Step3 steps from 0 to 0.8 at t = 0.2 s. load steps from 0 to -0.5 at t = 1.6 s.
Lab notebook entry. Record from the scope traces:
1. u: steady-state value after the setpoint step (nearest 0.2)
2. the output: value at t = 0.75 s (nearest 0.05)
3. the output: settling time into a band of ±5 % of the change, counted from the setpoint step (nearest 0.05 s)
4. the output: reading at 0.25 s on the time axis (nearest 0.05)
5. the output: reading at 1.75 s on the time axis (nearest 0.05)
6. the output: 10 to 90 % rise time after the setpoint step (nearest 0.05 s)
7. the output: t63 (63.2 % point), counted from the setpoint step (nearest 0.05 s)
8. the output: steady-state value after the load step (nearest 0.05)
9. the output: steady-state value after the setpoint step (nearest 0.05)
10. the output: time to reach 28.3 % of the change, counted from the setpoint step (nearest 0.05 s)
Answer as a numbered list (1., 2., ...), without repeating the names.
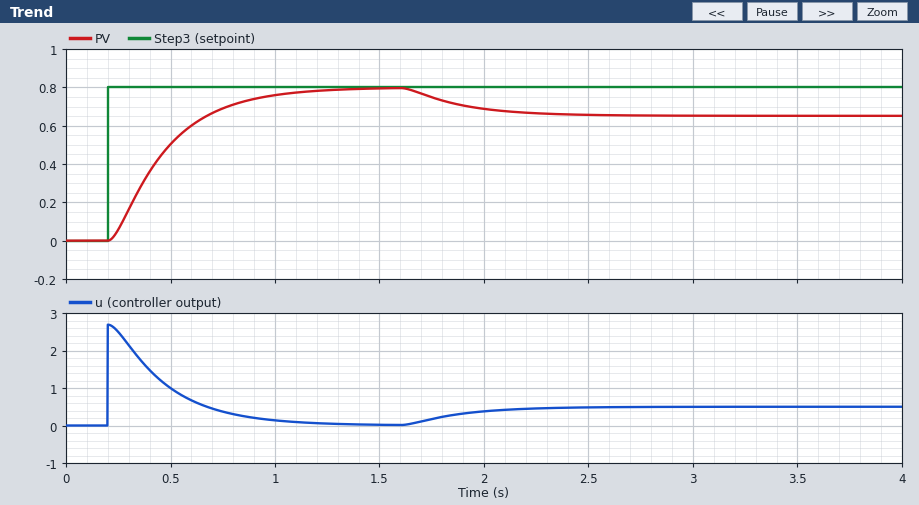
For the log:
1. 0.0
2. 0.70
3. 0.80 s
4. 0.05
5. 0.75
6. 0.55 s
7. 0.30 s
8. 0.65
9. 0.80
10. 0.15 s
